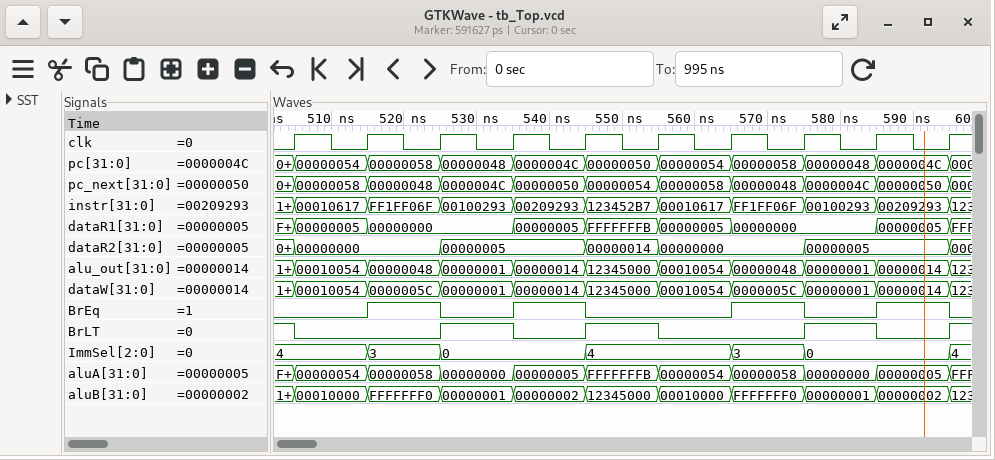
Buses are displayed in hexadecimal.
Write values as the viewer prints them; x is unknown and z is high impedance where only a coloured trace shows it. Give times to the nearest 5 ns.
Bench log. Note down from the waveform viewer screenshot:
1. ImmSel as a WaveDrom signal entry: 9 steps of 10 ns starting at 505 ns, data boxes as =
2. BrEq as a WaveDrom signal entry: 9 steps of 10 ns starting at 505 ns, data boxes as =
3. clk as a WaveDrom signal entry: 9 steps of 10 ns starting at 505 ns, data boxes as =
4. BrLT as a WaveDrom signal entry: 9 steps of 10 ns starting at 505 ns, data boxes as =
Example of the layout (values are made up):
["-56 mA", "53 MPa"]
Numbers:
["{name: 'ImmSel', wave: '===.=.==.', data: '4 3 0 4 3 0'}", "{name: 'BrEq', wave: '01010.101'}", "{name: 'clk', wave: 'p........'}", "{name: 'BrLT', wave: '0.1010.10'}"]
